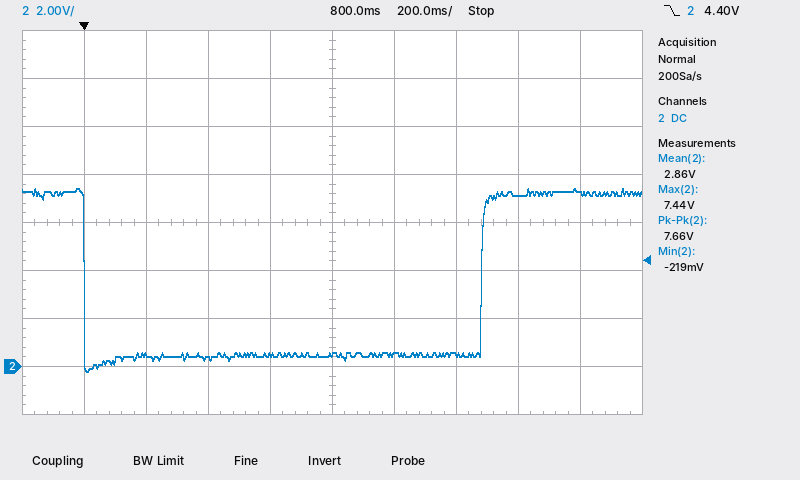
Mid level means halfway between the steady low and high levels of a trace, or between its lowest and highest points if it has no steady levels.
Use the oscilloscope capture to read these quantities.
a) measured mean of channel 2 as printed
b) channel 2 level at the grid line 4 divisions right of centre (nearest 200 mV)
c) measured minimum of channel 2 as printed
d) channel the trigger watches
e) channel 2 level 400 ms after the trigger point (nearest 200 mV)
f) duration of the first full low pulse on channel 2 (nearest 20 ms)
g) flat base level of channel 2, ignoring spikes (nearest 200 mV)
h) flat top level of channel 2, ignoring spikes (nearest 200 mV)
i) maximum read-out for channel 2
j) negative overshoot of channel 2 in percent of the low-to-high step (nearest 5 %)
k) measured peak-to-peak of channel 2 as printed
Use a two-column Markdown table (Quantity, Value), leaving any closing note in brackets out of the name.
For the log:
| Quantity | Value |
|---|---|
| measured mean of channel 2 as printed | 2.86 V |
| channel 2 level at the grid line 4 divisions right of centre | 7.2 V |
| measured minimum of channel 2 as printed | -219 mV |
| channel the trigger watches | channel 2 |
| channel 2 level 400 ms after the trigger point | 400 mV |
| duration of the first full low pulse on channel 2 | 1.28 s |
| flat base level of channel 2, ignoring spikes | 400 mV |
| flat top level of channel 2, ignoring spikes | 7.2 V |
| maximum read-out for channel 2 | 7.44 V |
| negative overshoot of channel 2 in percent of the low-to-high step | 10 % |
| measured peak-to-peak of channel 2 as printed | 7.66 V |
